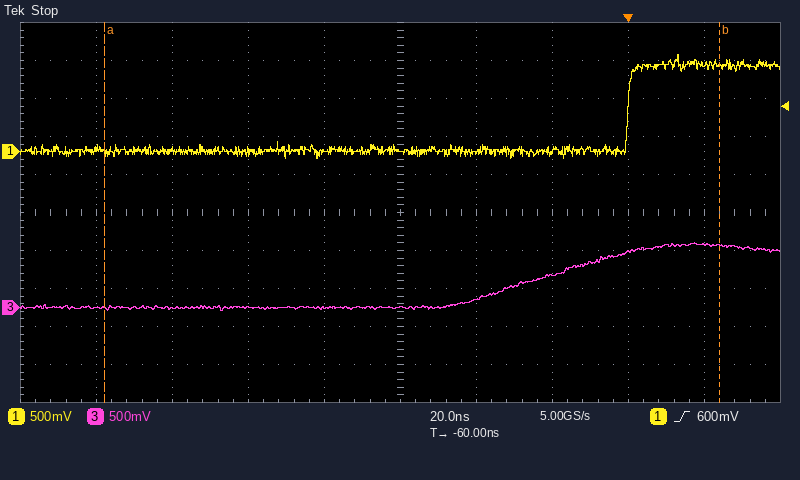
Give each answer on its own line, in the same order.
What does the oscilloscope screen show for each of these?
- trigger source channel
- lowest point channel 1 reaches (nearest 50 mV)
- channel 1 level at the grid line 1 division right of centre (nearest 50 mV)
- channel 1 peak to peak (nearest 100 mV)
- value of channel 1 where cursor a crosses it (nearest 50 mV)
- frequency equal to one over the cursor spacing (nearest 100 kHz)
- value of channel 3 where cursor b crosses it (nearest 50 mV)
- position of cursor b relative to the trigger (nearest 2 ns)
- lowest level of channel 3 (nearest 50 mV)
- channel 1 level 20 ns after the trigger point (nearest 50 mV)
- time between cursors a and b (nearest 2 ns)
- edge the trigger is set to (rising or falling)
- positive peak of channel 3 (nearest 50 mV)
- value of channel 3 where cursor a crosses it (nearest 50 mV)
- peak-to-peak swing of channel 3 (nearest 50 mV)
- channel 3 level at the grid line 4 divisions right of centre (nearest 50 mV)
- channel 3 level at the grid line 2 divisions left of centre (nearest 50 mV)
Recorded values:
channel 1
-100 mV
0 mV
1.40 V
0 mV
6.2 MHz
800 mV
+24 ns
-50 mV
1.15 V
162 ns
rising
850 mV
0 mV
900 mV
850 mV
0 mV
